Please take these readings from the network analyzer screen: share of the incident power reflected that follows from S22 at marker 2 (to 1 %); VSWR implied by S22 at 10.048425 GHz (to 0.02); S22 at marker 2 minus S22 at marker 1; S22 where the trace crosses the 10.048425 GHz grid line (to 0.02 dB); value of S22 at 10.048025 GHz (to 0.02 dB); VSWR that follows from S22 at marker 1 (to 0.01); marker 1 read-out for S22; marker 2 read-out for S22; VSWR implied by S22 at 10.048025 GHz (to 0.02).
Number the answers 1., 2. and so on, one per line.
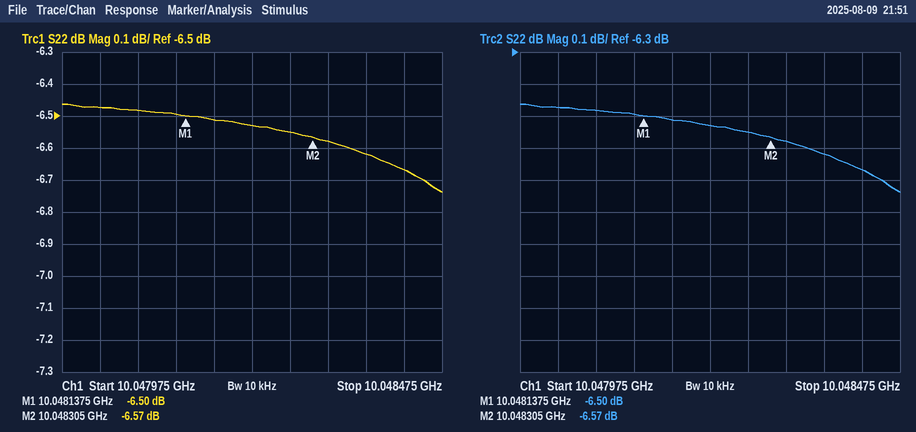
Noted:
1. 22 %
2. 2.74
3. -0.07 dB
4. -6.66 dB
5. -6.48 dB
6. 2.80
7. -6.50 dB
8. -6.57 dB
9. 2.80
